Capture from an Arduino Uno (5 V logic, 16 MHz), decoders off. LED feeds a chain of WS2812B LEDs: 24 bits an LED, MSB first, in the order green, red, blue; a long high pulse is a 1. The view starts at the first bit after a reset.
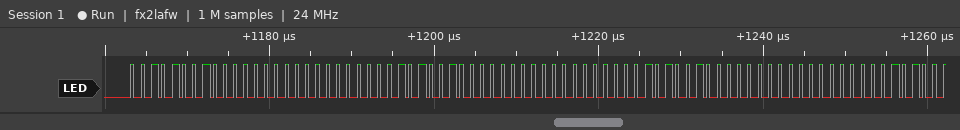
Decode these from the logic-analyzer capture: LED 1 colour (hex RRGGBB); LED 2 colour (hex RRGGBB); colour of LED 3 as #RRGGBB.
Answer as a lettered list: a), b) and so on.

a) #002900
b) #002900
c) #002900
